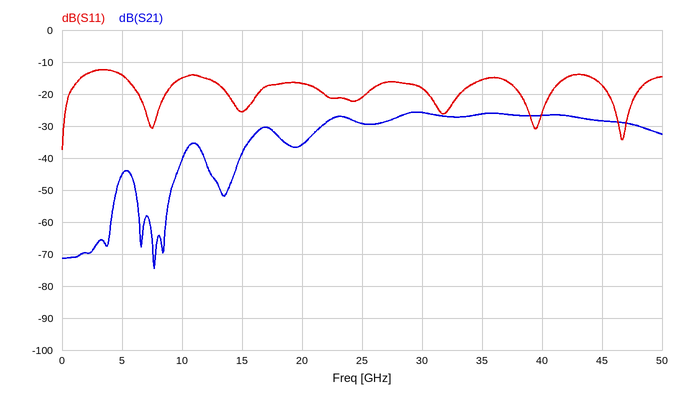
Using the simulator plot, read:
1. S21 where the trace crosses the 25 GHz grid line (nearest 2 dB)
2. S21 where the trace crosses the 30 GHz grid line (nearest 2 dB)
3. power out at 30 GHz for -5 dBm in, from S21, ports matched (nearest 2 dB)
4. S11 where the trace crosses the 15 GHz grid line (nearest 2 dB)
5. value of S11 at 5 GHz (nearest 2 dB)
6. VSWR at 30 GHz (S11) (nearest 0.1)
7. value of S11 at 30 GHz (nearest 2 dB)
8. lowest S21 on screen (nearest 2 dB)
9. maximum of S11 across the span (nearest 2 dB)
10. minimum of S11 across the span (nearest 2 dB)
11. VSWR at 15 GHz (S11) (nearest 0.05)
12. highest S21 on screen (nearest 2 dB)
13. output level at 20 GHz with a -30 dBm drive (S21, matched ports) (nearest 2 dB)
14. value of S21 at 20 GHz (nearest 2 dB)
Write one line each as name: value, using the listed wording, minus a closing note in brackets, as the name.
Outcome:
S21 where the trace crosses the 25 GHz grid line: -30 dB
S21 where the trace crosses the 30 GHz grid line: -26 dB
power out at 30 GHz for -5 dBm in, from S21, ports matched: -30 dBm
S11 where the trace crosses the 15 GHz grid line: -26 dB
value of S11 at 5 GHz: -14 dB
VSWR at 30 GHz (S11): 1.3
value of S11 at 30 GHz: -18 dB
lowest S21 on screen: -74 dB
maximum of S11 across the span: -12 dB
minimum of S11 across the span: -38 dB
VSWR at 15 GHz (S11): 1.10
highest S21 on screen: -26 dB
output level at 20 GHz with a -30 dBm drive (S21, matched ports): -66 dBm
value of S21 at 20 GHz: -36 dB
